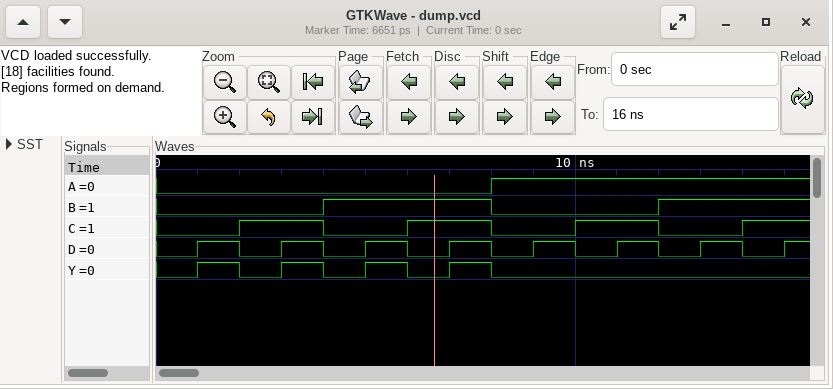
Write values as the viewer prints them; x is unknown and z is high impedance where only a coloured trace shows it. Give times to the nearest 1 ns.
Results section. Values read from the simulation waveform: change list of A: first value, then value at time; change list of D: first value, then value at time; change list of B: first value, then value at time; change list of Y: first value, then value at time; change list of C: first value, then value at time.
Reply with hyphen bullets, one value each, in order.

- 0, 1 at 8 ns
- 0, 1 at 1 ns, 0 at 2 ns, 1 at 3 ns, 0 at 4 ns, 1 at 5 ns, 0 at 6 ns, 1 at 7 ns, 0 at 8 ns, 1 at 9 ns, 0 at 10 ns, 1 at 11 ns, 0 at 12 ns, 1 at 13 ns, 0 at 14 ns, 1 at 15 ns
- 0, 1 at 4 ns, 0 at 8 ns, 1 at 12 ns
- 0, 1 at 1 ns, 0 at 2 ns, 1 at 3 ns, 0 at 4 ns, 1 at 5 ns, 0 at 6 ns, 1 at 7 ns, 0 at 8 ns
- 0, 1 at 2 ns, 0 at 4 ns, 1 at 6 ns, 0 at 8 ns, 1 at 10 ns, 0 at 12 ns, 1 at 14 ns
